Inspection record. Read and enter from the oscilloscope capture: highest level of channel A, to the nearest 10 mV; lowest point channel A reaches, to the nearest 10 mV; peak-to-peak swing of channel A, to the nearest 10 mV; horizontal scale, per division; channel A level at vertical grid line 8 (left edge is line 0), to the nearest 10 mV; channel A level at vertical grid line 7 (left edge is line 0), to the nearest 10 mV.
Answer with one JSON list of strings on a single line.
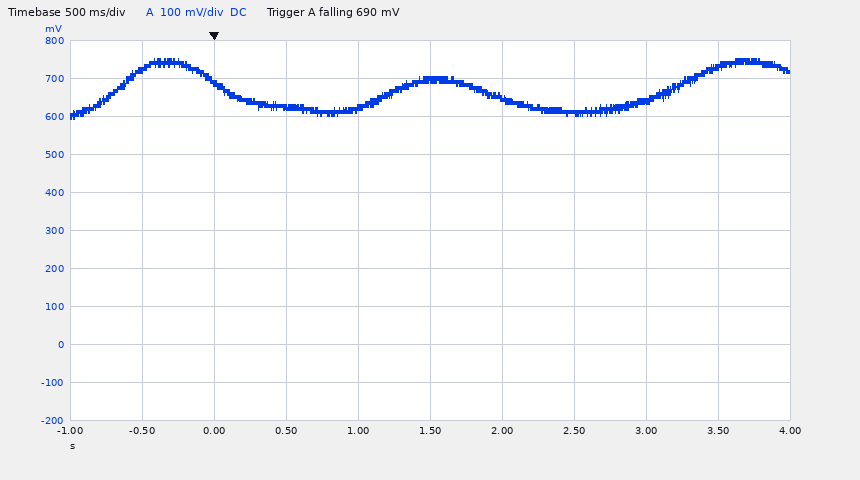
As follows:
["750 mV", "590 mV", "160 mV", "500 ms", "640 mV", "610 mV"]
